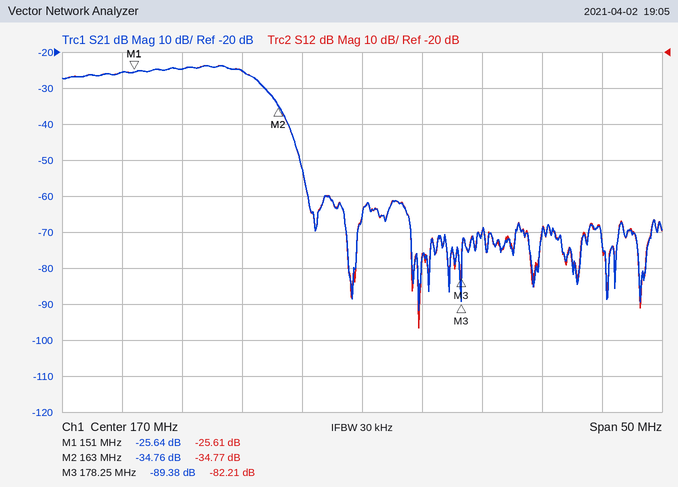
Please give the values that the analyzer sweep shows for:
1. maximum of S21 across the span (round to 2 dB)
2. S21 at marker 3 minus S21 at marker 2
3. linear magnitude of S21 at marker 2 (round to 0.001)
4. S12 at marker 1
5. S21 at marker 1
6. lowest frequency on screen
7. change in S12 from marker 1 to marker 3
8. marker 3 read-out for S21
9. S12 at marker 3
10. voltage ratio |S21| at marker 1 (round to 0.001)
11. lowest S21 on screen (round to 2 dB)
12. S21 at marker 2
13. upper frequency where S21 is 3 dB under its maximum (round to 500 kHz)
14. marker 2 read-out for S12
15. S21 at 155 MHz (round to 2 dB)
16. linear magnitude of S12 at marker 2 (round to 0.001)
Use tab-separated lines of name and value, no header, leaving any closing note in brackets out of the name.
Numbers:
maximum of S21 across the span	-24 dB
S21 at marker 3 minus S21 at marker 2	-54.62 dB
linear magnitude of S21 at marker 2	0.018
S12 at marker 1	-25.61 dB
S21 at marker 1	-25.64 dB
lowest frequency on screen	145 MHz
change in S12 from marker 1 to marker 3	-56.60 dB
marker 3 read-out for S21	-89.38 dB
S12 at marker 3	-82.21 dB
voltage ratio |S21| at marker 1	0.052
lowest S21 on screen	-92 dB
S21 at marker 2	-34.76 dB
upper frequency where S21 is 3 dB under its maximum	161.0 MHz
marker 2 read-out for S12	-34.77 dB
S21 at 155 MHz	-24 dB
linear magnitude of S12 at marker 2	0.018
